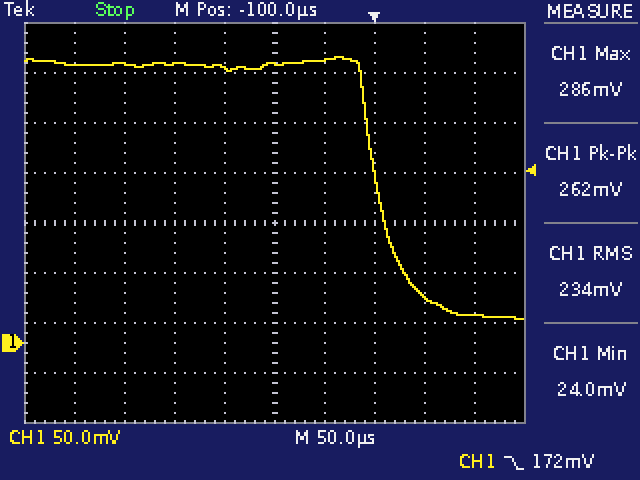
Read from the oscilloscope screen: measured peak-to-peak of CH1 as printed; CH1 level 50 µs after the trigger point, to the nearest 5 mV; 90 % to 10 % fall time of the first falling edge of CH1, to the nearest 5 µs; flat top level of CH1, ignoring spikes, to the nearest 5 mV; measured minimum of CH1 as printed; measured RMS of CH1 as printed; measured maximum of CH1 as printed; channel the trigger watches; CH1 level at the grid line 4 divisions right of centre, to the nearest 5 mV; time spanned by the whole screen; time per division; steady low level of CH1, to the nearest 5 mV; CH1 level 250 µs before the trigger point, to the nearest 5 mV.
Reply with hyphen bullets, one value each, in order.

- 262 mV
- 45 mV
- 55 µs
- 280 mV
- 24.0 mV
- 234 mV
- 286 mV
- CH1
- 30 mV
- 500 µs
- 50 µs
- 25 mV
- 280 mV
